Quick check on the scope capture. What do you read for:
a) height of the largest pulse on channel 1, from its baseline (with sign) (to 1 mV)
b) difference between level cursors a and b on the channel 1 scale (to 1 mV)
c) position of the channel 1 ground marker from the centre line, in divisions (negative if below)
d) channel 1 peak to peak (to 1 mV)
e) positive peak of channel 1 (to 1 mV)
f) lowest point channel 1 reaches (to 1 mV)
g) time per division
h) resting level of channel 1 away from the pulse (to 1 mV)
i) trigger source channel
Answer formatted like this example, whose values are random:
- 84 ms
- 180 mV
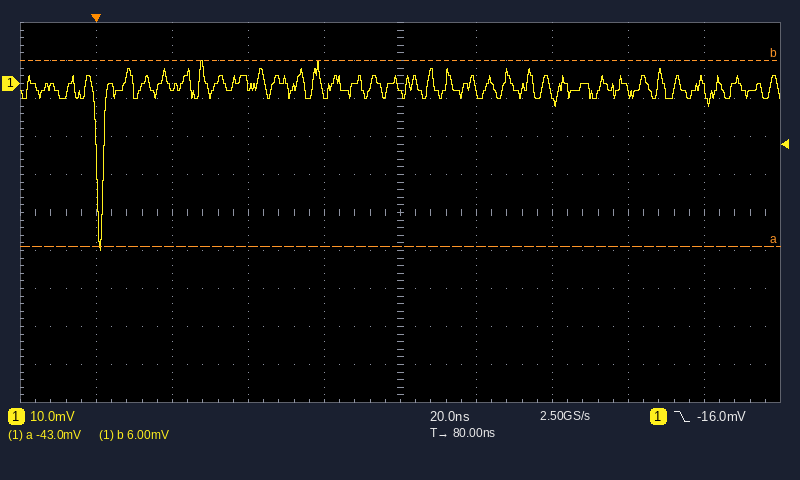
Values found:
- -43 mV
- 49 mV
- +3.4 div
- 50 mV
- 6 mV
- -44 mV
- 20 ns
- -1 mV
- channel 1
